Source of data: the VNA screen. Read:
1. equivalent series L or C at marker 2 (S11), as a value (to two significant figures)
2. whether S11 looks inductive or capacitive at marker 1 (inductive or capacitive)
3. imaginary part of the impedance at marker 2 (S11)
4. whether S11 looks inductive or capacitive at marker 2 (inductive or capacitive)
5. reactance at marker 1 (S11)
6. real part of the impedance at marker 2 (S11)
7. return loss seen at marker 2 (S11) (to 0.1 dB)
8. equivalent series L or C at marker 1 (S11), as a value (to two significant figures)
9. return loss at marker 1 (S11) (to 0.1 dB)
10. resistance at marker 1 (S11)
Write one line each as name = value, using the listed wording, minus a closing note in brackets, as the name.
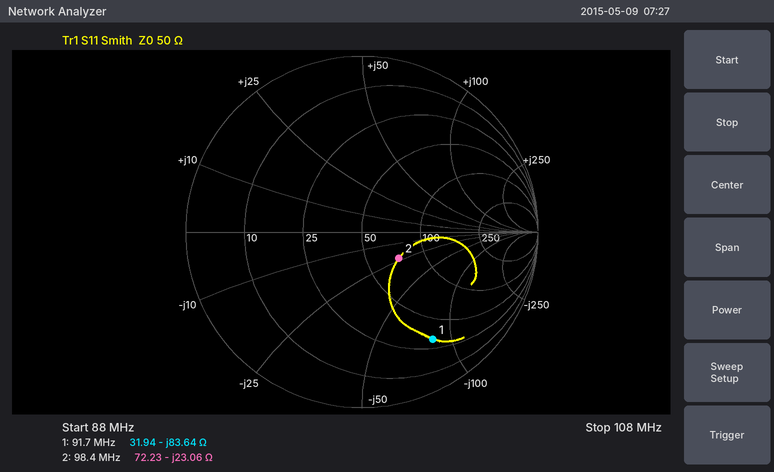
equivalent series L or C at marker 2 (S11), as a value = 70 pF
whether S11 looks inductive or capacitive at marker 1 = capacitive
imaginary part of the impedance at marker 2 = -23.06 Ω
whether S11 looks inductive or capacitive at marker 2 = capacitive
reactance at marker 1 = -83.64 Ω
real part of the impedance at marker 2 = 72.23 Ω
return loss seen at marker 2 (S11) = 11.8 dB
equivalent series L or C at marker 1 (S11), as a value = 21 pF
return loss at marker 1 (S11) = 2.7 dB
resistance at marker 1 = 31.94 Ω
